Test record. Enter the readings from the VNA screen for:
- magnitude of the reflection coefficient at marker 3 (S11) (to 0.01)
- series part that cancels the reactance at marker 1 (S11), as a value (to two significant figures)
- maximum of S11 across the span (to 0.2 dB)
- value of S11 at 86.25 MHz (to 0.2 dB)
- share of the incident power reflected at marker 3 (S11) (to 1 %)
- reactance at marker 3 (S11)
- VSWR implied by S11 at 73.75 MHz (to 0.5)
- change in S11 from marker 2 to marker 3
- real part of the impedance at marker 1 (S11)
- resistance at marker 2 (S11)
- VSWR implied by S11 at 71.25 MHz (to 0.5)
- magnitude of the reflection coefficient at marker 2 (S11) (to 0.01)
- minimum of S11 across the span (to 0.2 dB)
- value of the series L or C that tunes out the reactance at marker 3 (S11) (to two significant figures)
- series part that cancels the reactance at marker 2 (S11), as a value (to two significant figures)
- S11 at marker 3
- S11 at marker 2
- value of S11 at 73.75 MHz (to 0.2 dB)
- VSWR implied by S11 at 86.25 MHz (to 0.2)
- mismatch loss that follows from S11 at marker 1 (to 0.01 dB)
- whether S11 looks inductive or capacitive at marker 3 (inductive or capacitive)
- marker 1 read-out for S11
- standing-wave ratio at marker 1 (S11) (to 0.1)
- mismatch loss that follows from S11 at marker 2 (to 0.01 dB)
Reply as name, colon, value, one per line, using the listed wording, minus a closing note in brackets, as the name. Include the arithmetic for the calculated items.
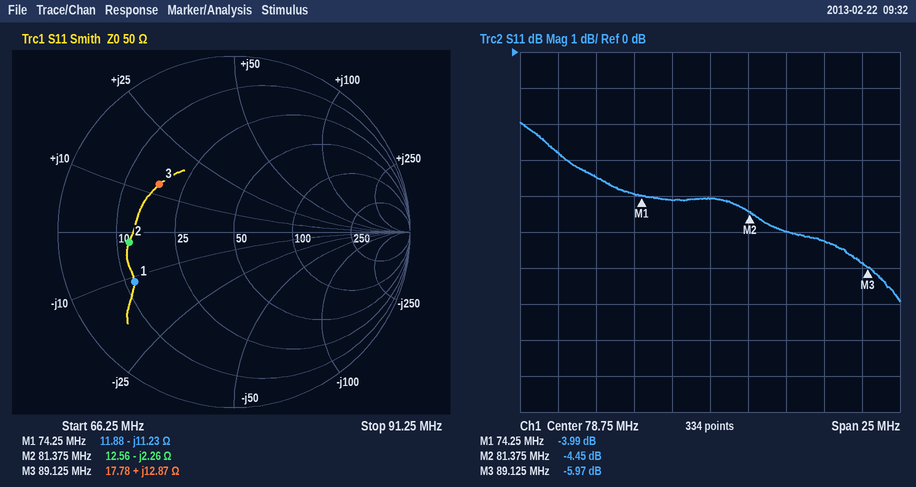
magnitude of the reflection coefficient at marker 3 (S11): 0.50
series part that cancels the reactance at marker 1 (S11), as a value: L = 11.23 Ω/(2π × 74.25 MHz) ≈ 24 nH
maximum of S11 across the span: -2.0 dB
value of S11 at 86.25 MHz: -5.2 dB
share of the incident power reflected at marker 3 (S11): 10^(-5.97/10) ≈ 25 %
reactance at marker 3: +12.87 Ω
VSWR implied by S11 at 73.75 MHz: |Γ| = 10^(-4/20) = 0.6310; VSWR = (1 + 0.6310)/(1 − 0.6310) ≈ 4.42, so 4.5 to the nearest 0.5
change in S11 from marker 2 to marker 3: -5.97 − (-4.45) = -1.52 dB
real part of the impedance at marker 1: 11.88 Ω
resistance at marker 2: 12.56 Ω
VSWR implied by S11 at 71.25 MHz: |Γ| = 10^(-3.4/20) = 0.6761; VSWR = (1 + 0.6761)/(1 − 0.6761) ≈ 5.17, so 5.0 to the nearest 0.5
magnitude of the reflection coefficient at marker 2 (S11): 0.60
minimum of S11 across the span: -7.0 dB
value of the series L or C that tunes out the reactance at marker 3 (S11): C = 1/(2π × 89.125 MHz × 12.87 Ω) ≈ 139 pF, so 140 pF to two significant figures
series part that cancels the reactance at marker 2 (S11), as a value: L = 2.26 Ω/(2π × 81.375 MHz) ≈ 4.4 nH
S11 at marker 3: -5.97 dB
S11 at marker 2: -4.45 dB
value of S11 at 73.75 MHz: -4.0 dB
VSWR implied by S11 at 86.25 MHz: |Γ| = 10^(-5.2/20) = 0.5495; VSWR = (1 + 0.5495)/(1 − 0.5495) ≈ 3.4
mismatch loss that follows from S11 at marker 1: −10 log10(1 − 10^(-3.99/10)) ≈ 2.21 dB
whether S11 looks inductive or capacitive at marker 3: inductive
marker 1 read-out for S11: -3.99 dB
standing-wave ratio at marker 1 (S11): 4.4
mismatch loss that follows from S11 at marker 2: −10 log10(1 − 10^(-4.45/10)) ≈ 1.93 dB
